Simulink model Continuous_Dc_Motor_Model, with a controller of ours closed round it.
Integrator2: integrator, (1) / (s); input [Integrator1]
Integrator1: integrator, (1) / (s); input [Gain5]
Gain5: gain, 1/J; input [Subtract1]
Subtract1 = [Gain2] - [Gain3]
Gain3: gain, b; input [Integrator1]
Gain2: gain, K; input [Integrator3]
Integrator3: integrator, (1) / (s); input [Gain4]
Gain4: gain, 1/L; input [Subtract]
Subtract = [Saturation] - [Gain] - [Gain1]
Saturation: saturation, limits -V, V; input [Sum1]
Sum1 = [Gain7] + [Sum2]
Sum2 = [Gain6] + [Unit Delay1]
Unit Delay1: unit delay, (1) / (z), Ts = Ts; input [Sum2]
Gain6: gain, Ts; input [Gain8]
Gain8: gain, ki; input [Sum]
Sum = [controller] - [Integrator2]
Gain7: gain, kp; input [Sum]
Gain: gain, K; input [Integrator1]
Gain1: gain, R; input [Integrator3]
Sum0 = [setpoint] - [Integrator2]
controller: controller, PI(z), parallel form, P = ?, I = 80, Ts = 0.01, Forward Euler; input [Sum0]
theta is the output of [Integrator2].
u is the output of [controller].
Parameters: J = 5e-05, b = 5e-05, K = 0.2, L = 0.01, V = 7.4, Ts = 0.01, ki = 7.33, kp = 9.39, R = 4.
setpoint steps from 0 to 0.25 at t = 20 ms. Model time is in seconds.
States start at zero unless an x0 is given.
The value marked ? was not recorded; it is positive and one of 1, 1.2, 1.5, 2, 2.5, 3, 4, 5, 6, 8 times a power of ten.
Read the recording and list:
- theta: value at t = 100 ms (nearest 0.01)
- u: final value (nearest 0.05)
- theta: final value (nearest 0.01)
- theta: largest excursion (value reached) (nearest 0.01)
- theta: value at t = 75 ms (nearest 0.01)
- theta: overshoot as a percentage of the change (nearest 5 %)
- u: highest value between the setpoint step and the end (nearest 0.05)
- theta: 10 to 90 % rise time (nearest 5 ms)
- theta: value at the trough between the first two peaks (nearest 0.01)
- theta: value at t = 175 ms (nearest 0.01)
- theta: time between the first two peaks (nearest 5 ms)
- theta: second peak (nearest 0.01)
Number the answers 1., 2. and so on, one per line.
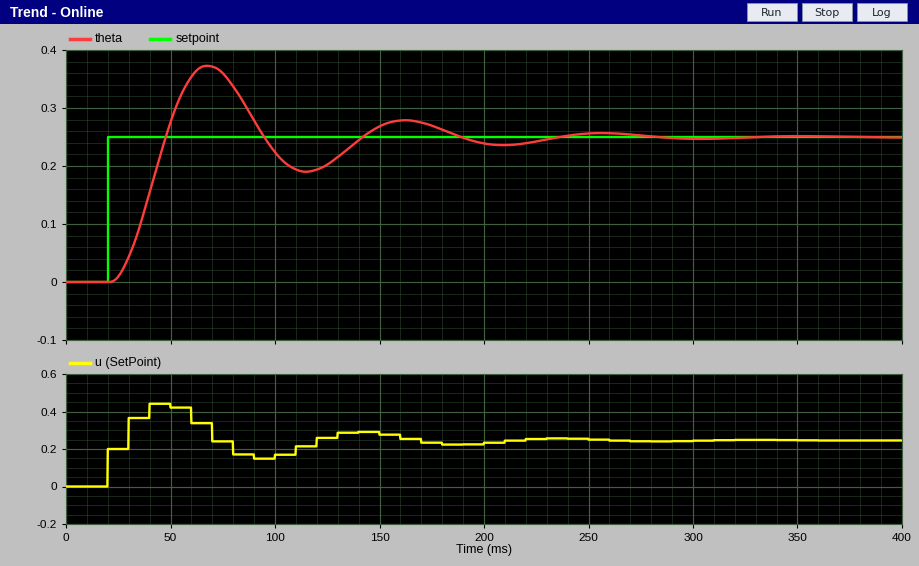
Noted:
1. 0.22
2. 0.25
3. 0.25
4. 0.37
5. 0.36
6. 50 %
7. 0.45
8. 20 ms
9. 0.19
10. 0.27
11. 95 ms
12. 0.28
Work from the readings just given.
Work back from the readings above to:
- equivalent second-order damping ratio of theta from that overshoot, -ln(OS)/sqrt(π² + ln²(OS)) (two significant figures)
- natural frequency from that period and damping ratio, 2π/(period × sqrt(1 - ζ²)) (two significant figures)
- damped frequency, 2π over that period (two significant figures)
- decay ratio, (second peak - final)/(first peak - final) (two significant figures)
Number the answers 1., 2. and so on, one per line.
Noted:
1. 0.22
2. 0.068 rad/ms
3. 0.066 rad/ms
4. 0.25
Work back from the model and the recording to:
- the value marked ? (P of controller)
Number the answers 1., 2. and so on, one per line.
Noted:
1. 0.8
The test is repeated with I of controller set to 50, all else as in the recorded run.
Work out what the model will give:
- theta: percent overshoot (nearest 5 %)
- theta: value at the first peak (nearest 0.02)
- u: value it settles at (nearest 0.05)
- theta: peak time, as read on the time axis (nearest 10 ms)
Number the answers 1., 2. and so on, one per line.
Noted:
1. 15 %
2. 0.28
3. 0.25
4. 70 ms
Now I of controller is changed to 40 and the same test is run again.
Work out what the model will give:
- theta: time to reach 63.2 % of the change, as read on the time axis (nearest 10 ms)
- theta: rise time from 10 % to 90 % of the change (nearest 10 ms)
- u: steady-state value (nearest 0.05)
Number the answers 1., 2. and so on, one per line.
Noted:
1. 40 ms
2. 30 ms
3. 0.25
